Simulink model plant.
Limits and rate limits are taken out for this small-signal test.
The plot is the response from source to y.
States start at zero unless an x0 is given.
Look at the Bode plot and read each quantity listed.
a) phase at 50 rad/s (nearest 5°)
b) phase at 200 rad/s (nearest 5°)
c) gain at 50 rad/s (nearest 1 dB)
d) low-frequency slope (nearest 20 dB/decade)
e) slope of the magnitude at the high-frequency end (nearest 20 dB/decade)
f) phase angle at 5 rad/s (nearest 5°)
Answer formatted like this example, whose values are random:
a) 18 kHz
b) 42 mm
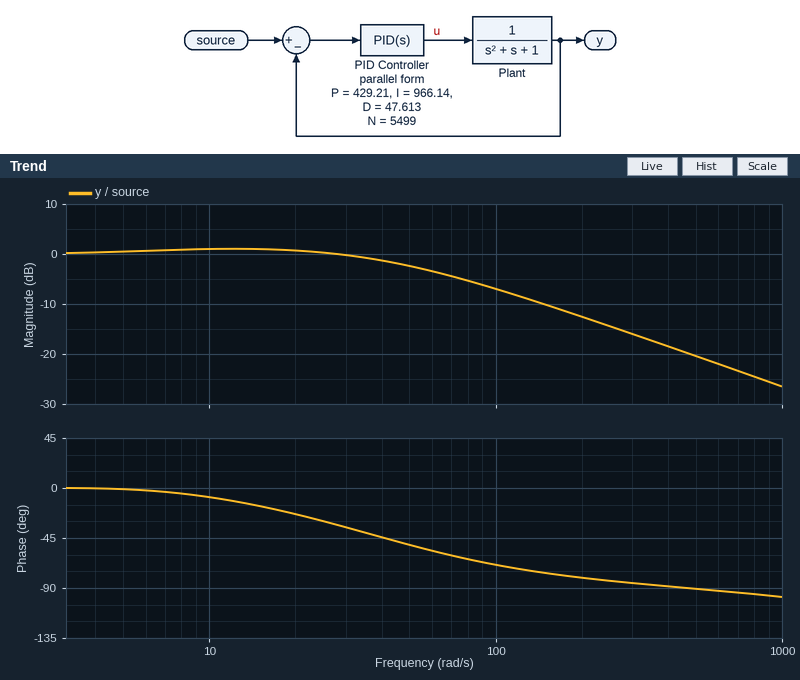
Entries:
a) -50°
b) -80°
c) -2 dB
d) 0 dB/decade
e) -20 dB/decade
f) 0°
